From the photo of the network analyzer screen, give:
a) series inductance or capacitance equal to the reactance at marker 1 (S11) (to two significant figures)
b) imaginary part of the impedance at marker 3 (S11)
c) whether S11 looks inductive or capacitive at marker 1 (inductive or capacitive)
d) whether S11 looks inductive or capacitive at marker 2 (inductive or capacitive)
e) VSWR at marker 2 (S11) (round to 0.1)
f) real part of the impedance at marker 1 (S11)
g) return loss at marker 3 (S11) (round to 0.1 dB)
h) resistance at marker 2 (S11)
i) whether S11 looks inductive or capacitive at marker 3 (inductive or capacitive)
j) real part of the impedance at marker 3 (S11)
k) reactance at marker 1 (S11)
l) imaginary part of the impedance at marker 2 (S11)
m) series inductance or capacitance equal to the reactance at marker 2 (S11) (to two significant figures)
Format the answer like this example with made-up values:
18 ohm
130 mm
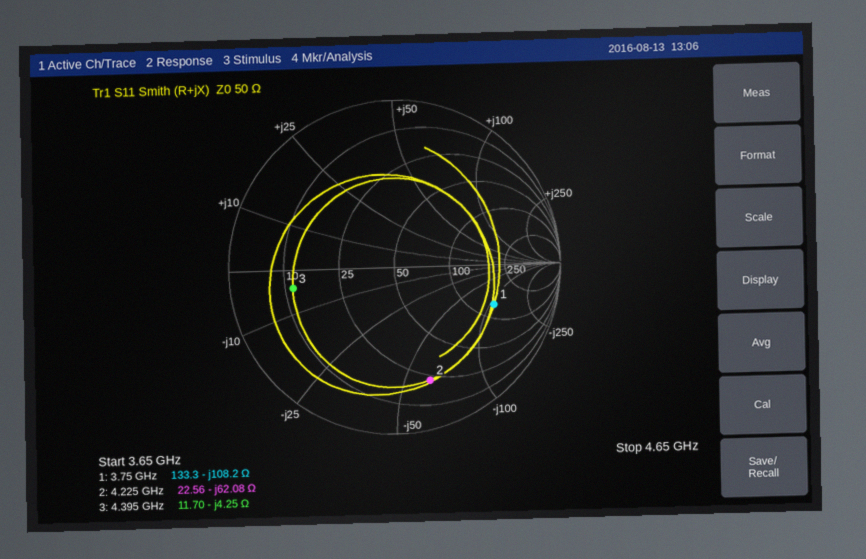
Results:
390 fF
-4.25 Ω
capacitive
capacitive
5.9
133.3 Ω
4.1 dB
22.56 Ω
capacitive
11.70 Ω
-108.2 Ω
-62.08 Ω
610 fF
